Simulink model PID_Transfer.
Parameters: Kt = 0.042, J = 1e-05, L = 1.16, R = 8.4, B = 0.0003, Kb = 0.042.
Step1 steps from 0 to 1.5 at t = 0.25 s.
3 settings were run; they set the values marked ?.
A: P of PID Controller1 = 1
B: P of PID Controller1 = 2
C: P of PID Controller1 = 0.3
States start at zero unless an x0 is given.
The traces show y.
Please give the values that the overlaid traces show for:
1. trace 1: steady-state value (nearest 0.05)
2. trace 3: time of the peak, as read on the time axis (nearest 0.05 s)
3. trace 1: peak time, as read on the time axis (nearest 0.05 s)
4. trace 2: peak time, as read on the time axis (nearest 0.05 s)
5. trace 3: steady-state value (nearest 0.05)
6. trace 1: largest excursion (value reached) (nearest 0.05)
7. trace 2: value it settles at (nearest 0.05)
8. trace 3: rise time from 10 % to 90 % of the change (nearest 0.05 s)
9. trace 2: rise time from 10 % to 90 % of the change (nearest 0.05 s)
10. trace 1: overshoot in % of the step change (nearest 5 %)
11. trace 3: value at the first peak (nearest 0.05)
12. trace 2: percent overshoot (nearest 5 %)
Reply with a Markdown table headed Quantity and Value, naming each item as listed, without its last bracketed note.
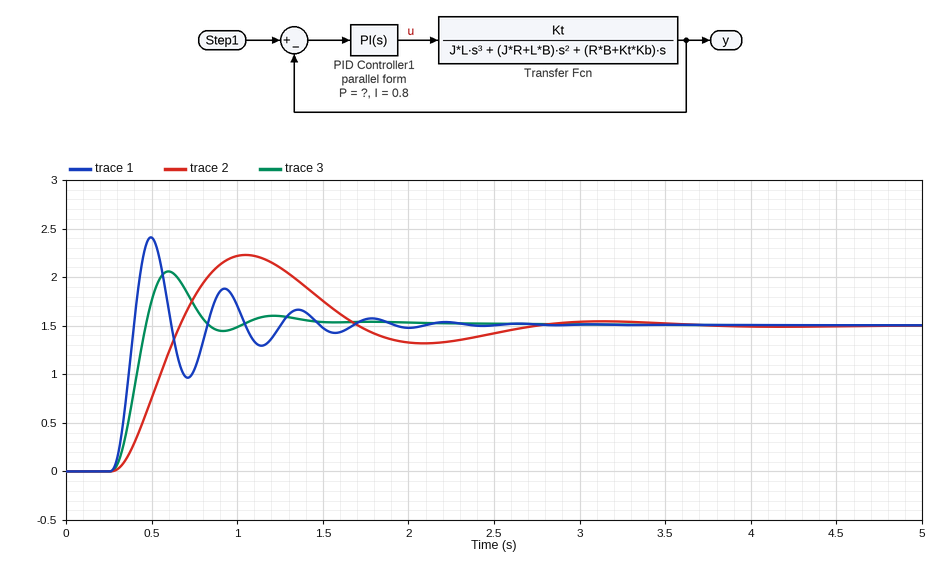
| Quantity | Value |
|---|---|
| trace 1: steady-state value | 1.50 |
| trace 3: time of the peak, as read on the time axis | 0.60 s |
| trace 1: peak time, as read on the time axis | 0.50 s |
| trace 2: peak time, as read on the time axis | 1.05 s |
| trace 3: steady-state value | 1.50 |
| trace 1: largest excursion (value reached) | 2.40 |
| trace 2: value it settles at | 1.50 |
| trace 3: rise time from 10 % to 90 % of the change | 0.15 s |
| trace 2: rise time from 10 % to 90 % of the change | 0.25 s |
| trace 1: overshoot in % of the step change | 60 % |
| trace 3: value at the first peak | 2.05 |
| trace 2: percent overshoot | 50 % |
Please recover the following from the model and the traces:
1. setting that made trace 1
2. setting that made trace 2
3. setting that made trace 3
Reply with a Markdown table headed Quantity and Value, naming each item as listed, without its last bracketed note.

| Quantity | Value |
|---|---|
| setting that made trace 1 | B |
| setting that made trace 2 | C |
| setting that made trace 3 | A |
